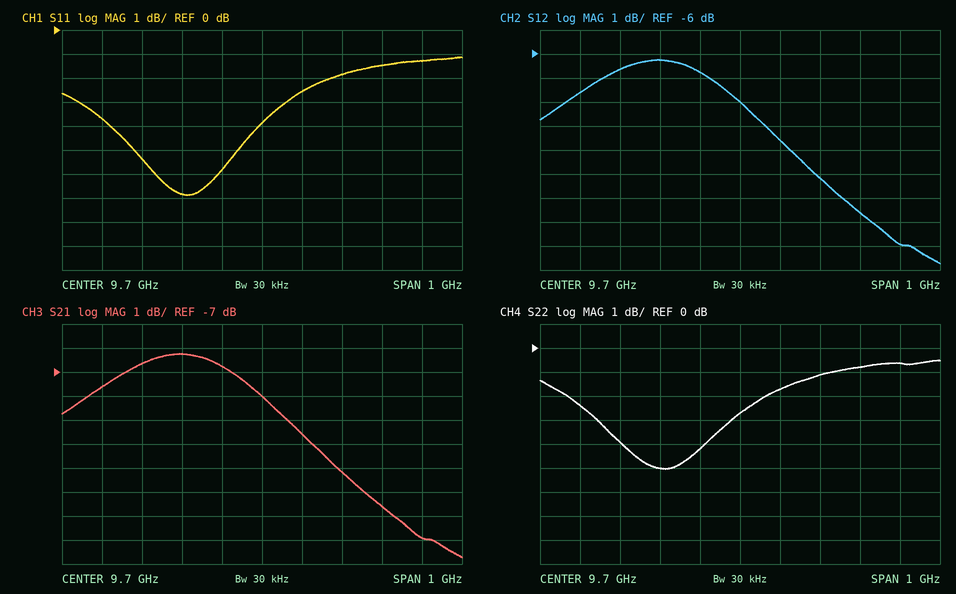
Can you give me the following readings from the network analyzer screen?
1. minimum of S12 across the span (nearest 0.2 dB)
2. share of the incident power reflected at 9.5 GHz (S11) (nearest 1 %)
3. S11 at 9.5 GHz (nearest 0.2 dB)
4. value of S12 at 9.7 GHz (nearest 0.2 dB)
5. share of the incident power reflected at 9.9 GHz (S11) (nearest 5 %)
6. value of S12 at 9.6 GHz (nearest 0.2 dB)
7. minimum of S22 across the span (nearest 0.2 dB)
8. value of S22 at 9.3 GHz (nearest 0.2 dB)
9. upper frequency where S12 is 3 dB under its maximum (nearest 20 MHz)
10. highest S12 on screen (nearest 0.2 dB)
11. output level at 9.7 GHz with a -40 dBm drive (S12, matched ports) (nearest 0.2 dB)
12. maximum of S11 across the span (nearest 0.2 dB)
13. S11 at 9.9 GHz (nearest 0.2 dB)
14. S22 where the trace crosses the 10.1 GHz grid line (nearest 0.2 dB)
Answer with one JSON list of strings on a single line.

["-14.8 dB", "21 %", "-6.8 dB", "-8.0 dB", "65 %", "-6.8 dB", "-5.0 dB", "-2.4 dB", "9.78 GHz", "-6.2 dB", "-48.0 dBm", "-1.2 dB", "-1.8 dB", "-0.6 dB"]
